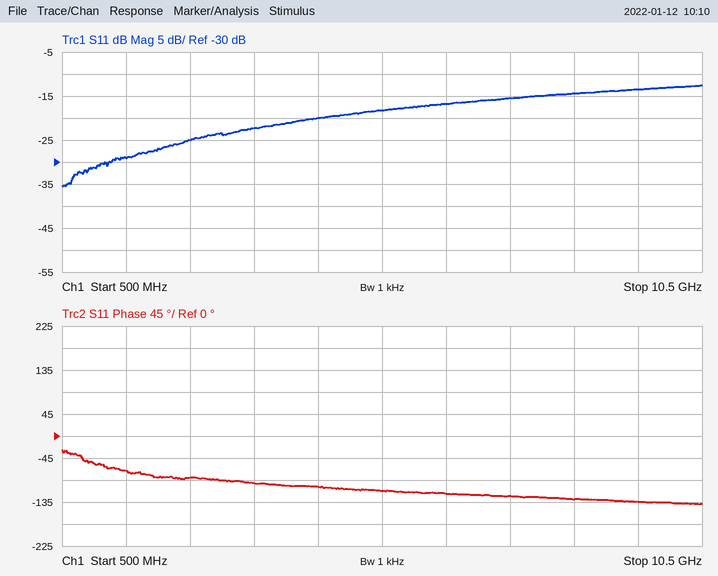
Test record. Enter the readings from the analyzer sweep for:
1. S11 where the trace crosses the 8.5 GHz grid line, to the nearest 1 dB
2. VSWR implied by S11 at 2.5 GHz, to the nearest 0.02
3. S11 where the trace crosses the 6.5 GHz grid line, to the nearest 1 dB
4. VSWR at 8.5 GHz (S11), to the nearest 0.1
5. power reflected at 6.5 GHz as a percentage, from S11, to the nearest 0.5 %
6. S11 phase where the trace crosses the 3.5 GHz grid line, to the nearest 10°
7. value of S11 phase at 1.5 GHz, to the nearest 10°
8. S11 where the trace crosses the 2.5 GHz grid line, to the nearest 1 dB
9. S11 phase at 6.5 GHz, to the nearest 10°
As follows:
-14 dB
1.12
-17 dB
1.5
2.0 %
-100°
-70°
-25 dB
-120°
